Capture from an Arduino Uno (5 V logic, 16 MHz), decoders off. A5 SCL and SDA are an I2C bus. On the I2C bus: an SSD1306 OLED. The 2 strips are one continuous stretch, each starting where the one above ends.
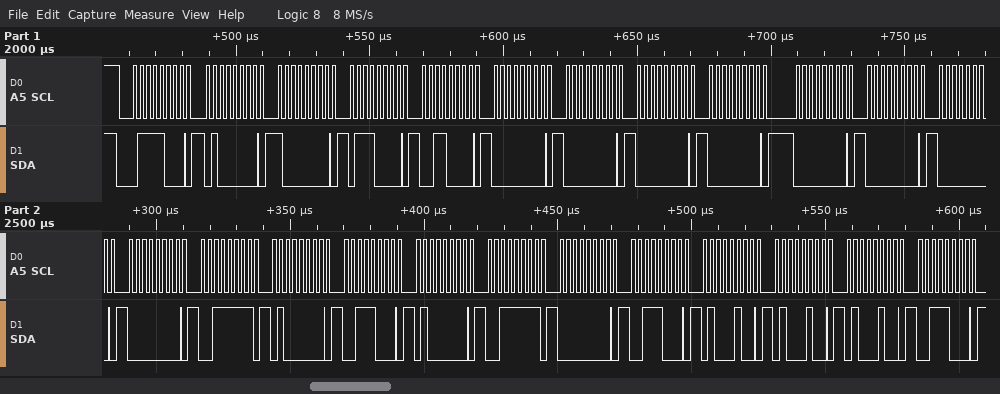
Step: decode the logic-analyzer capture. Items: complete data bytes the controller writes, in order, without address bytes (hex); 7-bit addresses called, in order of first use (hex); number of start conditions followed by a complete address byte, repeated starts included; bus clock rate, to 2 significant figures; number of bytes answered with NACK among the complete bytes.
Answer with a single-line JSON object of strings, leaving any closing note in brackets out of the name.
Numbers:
{"complete data bytes the controller writes, in order, without address bytes": "40 80 70 30 00 00 00 00 00 00 00 00 3F 40 38 40 3F 00 38 44 44 44 38", "7-bit addresses called, in order of first use": "0x3C", "number of start conditions followed by a complete address byte, repeated starts included": "1", "bus clock rate, to 2 significant figures": "400 kHz", "number of bytes answered with NACK among the complete bytes": "0"}
